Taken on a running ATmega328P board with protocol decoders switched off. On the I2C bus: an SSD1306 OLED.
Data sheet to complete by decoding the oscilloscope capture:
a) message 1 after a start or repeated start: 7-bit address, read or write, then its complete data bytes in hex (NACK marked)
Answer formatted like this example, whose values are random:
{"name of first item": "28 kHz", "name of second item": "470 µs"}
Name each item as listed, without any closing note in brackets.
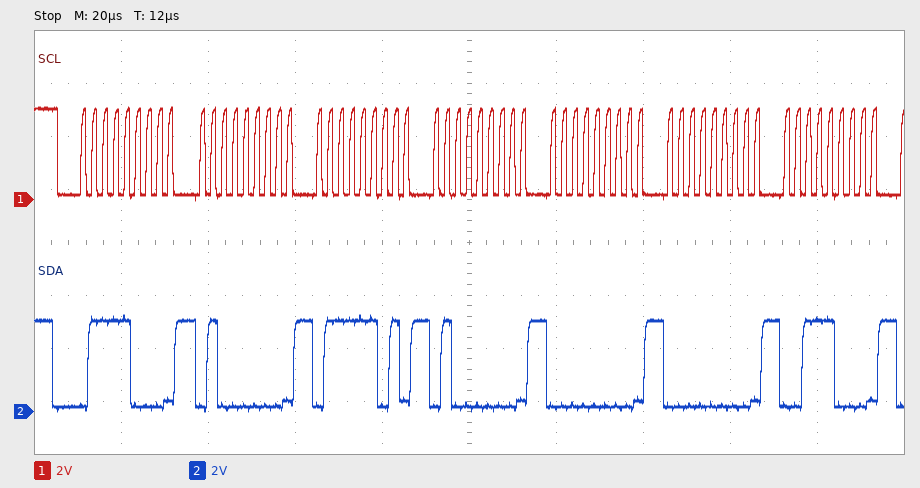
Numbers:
{"message 1 after a start or repeated start: 7-bit address, read or write, then its complete data bytes in hex": "0x3C write: 40 7D 40 00 00 38"}
